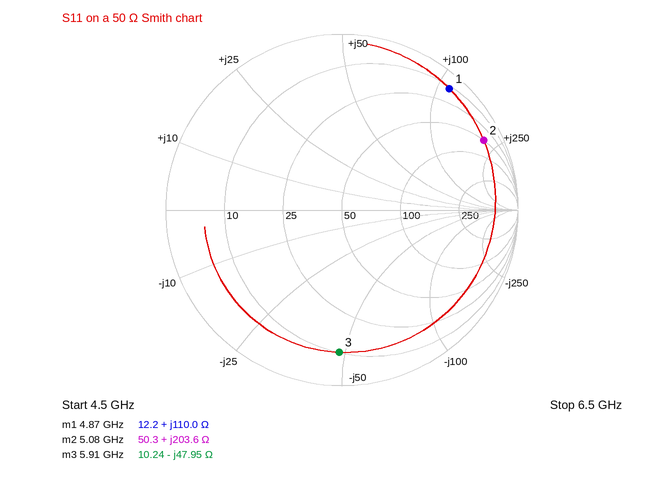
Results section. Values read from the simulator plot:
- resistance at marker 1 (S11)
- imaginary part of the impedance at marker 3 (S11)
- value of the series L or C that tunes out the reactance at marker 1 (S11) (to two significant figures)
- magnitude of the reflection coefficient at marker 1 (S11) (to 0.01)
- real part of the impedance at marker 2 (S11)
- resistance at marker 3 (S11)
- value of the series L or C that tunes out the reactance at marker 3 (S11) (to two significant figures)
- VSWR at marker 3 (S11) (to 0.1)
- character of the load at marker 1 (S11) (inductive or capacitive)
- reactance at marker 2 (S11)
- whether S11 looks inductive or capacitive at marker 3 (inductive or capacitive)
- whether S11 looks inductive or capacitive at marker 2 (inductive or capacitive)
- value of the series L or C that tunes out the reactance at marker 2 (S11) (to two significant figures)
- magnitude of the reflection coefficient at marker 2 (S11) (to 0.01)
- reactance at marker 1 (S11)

12.2 Ω
-47.95 Ω
300 fF
0.92
50.3 Ω
10.24 Ω
1.3 nH
9.5
inductive
+203.6 Ω
capacitive
inductive
150 fF
0.90
+110.0 Ω
